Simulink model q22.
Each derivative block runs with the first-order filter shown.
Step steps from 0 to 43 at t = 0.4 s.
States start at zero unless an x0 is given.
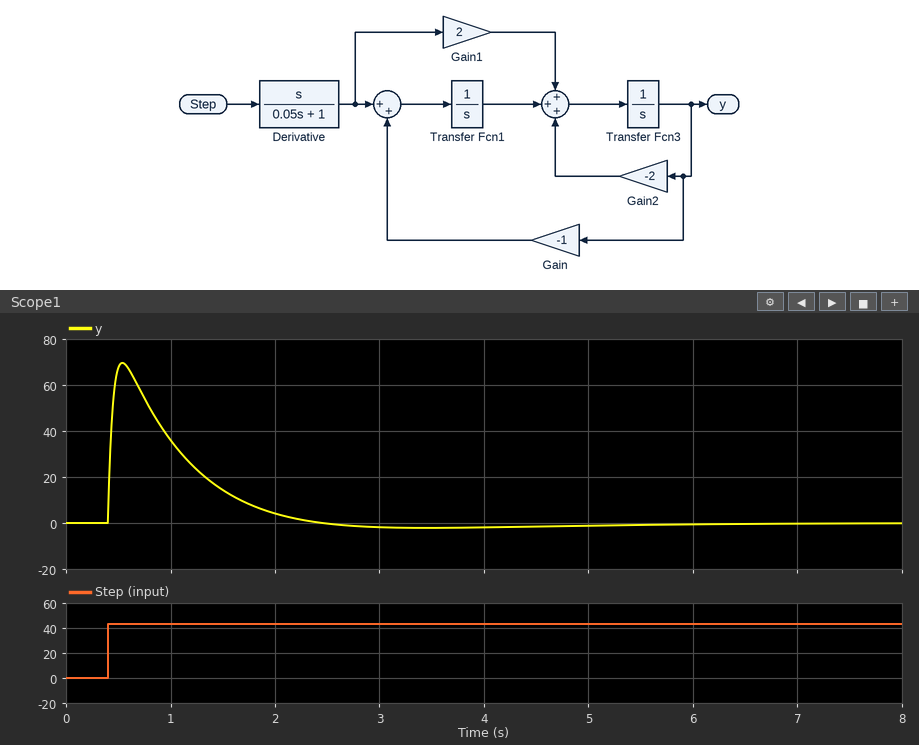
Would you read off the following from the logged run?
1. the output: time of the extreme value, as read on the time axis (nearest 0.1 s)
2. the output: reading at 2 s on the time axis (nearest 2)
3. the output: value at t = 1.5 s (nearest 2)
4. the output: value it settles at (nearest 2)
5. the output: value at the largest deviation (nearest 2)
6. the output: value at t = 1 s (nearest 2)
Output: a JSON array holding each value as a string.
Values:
["0.5 s", "4", "14", "0", "70", "36"]
